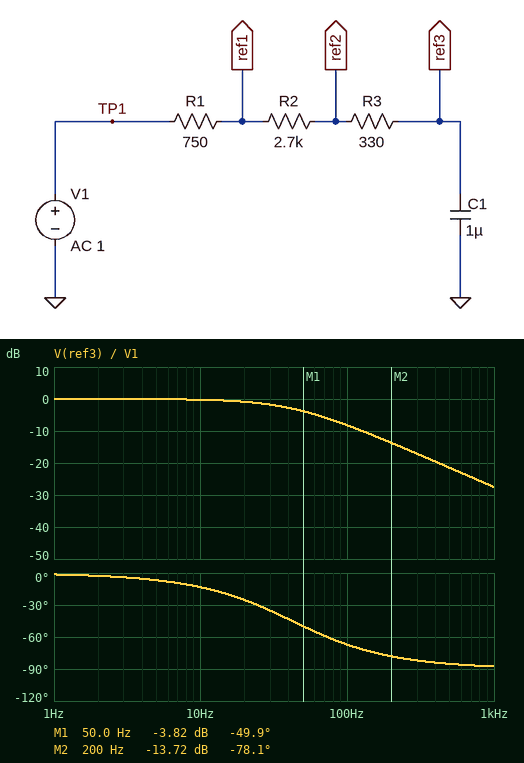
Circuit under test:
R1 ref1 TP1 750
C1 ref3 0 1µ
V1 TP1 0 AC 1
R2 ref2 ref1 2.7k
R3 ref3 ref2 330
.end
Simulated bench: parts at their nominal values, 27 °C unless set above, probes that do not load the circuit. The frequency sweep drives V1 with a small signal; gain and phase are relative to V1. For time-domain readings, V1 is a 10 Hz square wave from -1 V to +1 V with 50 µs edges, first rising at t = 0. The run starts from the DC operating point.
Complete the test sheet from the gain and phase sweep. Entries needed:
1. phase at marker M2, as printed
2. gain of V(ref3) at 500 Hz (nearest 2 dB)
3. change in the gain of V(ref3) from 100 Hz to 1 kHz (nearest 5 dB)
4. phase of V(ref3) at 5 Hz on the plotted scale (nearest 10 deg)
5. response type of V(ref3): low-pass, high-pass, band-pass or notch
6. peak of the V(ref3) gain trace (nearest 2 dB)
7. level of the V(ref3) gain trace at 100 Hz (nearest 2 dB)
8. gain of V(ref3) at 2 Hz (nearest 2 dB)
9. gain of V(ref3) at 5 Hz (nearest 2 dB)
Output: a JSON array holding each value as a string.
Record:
["-78.1 deg", "-22 dB", "-20 dB", "-10 deg", "low-pass", "0 dB", "-8 dB", "0 dB", "0 dB"]
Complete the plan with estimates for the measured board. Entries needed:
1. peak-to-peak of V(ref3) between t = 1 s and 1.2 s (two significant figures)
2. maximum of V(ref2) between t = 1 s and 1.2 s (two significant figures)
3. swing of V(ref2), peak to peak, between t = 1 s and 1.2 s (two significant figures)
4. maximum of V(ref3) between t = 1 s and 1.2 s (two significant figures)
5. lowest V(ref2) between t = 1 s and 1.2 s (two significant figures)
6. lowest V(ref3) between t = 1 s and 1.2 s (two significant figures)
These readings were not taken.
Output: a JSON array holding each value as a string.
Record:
["2.0 V", "1.0 V", "2.0 V", "1.0 V", "-1.0 V", "-1.0 V"]
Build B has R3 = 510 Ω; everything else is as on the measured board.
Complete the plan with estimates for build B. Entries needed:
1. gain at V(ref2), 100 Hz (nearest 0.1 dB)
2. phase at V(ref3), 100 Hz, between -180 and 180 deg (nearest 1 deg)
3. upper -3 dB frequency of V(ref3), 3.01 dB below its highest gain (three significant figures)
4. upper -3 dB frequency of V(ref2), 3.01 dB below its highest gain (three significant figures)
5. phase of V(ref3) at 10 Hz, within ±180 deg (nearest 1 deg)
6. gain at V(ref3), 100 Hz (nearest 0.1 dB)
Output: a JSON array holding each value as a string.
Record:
["-8.1 dB", "-68 deg", "40.2 Hz", "40.9 Hz", "-14 deg", "-8.6 dB"]
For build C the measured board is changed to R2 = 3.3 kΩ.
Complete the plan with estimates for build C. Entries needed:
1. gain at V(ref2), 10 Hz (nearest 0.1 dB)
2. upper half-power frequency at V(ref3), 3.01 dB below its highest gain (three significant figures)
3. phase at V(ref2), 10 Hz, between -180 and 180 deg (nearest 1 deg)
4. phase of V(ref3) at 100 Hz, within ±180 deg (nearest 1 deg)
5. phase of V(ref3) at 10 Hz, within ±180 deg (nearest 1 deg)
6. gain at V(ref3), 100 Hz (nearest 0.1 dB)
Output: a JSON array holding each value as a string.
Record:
["-0.3 dB", "36.3 Hz", "-14 deg", "-70 deg", "-15 deg", "-9.3 dB"]
